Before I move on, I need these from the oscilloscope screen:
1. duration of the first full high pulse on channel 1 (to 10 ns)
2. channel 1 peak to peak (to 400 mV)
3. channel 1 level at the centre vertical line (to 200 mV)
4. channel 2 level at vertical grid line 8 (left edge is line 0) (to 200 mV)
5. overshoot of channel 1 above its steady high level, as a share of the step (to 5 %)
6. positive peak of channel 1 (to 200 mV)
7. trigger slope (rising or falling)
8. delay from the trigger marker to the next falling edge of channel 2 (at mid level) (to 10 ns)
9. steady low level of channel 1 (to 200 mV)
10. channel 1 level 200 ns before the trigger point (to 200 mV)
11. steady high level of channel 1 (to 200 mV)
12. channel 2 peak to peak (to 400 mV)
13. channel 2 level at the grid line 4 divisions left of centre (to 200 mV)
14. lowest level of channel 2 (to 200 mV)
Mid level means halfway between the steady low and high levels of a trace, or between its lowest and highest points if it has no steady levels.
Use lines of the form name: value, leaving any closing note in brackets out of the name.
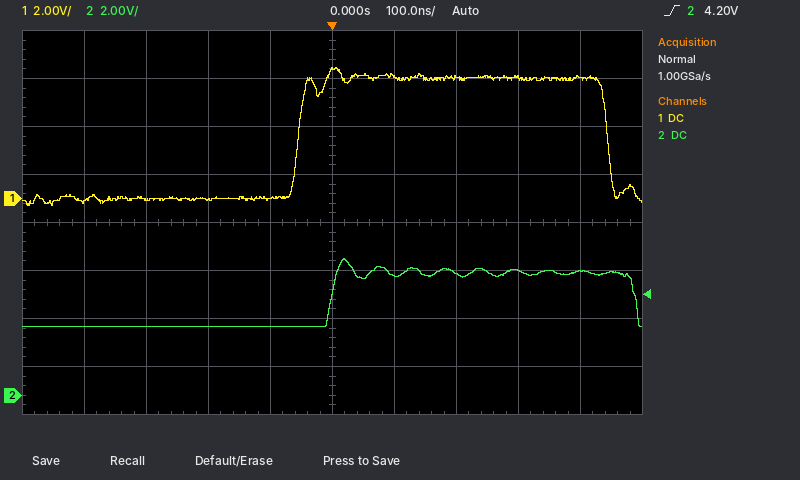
duration of the first full high pulse on channel 1: 500 ns
channel 1 peak to peak: 5.6 V
channel 1 level at the centre vertical line: 5.4 V
channel 2 level at vertical grid line 8 (left edge is line 0): 5.2 V
overshoot of channel 1 above its steady high level, as a share of the step: 10 %
positive peak of channel 1: 5.4 V
trigger slope: rising
delay from the trigger marker to the next falling edge of channel 2 (at mid level): 490 ns
steady low level of channel 1: 0.0 V
channel 1 level 200 ns before the trigger point: 0.0 V
steady high level of channel 1: 5.0 V
channel 2 peak to peak: 2.8 V
channel 2 level at the grid line 4 divisions left of centre: 2.8 V
lowest level of channel 2: 2.8 V
